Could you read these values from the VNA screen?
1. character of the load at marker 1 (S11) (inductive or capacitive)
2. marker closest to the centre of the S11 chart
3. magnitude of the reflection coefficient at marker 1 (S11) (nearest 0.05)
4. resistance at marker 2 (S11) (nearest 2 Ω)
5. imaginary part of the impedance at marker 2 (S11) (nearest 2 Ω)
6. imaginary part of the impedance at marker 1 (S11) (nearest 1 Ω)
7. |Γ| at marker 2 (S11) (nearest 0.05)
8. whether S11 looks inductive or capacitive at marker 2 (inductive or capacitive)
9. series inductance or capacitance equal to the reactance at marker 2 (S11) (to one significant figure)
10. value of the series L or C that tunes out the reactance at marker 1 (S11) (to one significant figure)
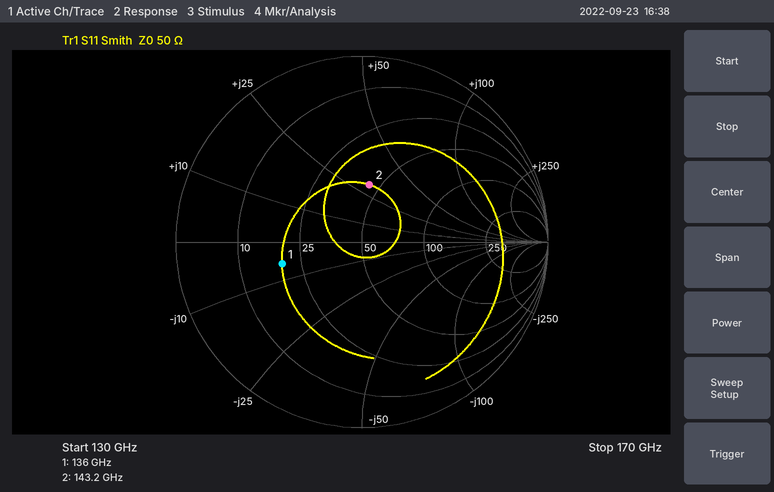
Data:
capacitive
marker 2
0.45
44 Ω
+30 Ω
-6 Ω
0.30
inductive
30 pH
7 pH
